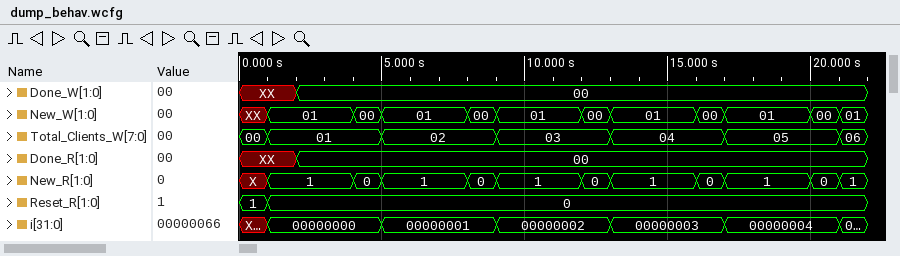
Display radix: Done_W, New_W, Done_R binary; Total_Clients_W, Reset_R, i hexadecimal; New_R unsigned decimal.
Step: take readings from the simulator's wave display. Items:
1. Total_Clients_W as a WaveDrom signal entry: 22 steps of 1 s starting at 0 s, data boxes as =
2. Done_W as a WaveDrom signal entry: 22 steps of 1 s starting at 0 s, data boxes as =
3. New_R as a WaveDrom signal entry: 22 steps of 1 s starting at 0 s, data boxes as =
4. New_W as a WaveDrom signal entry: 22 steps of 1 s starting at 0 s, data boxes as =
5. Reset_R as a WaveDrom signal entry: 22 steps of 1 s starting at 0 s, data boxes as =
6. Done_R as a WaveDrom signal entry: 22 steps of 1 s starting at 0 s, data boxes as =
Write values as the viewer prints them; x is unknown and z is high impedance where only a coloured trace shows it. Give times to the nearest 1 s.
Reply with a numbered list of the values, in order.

1. {name: 'Total_Clients_W', wave: '==...=...=...=...=...=', data: '00 01 02 03 04 05 06'}
2. {name: 'Done_W', wave: 'x.=...................', data: '00'}
3. {name: 'New_R', wave: 'x=..==..==..==..==..==', data: '1 0 1 0 1 0 1 0 1 0 1'}
4. {name: 'New_W', wave: 'x=..==..==..==..==..==', data: '01 00 01 00 01 00 01 00 01 00 01'}
5. {name: 'Reset_R', wave: '==....................', data: '1 0'}
6. {name: 'Done_R', wave: 'x.=...................', data: '00'}
